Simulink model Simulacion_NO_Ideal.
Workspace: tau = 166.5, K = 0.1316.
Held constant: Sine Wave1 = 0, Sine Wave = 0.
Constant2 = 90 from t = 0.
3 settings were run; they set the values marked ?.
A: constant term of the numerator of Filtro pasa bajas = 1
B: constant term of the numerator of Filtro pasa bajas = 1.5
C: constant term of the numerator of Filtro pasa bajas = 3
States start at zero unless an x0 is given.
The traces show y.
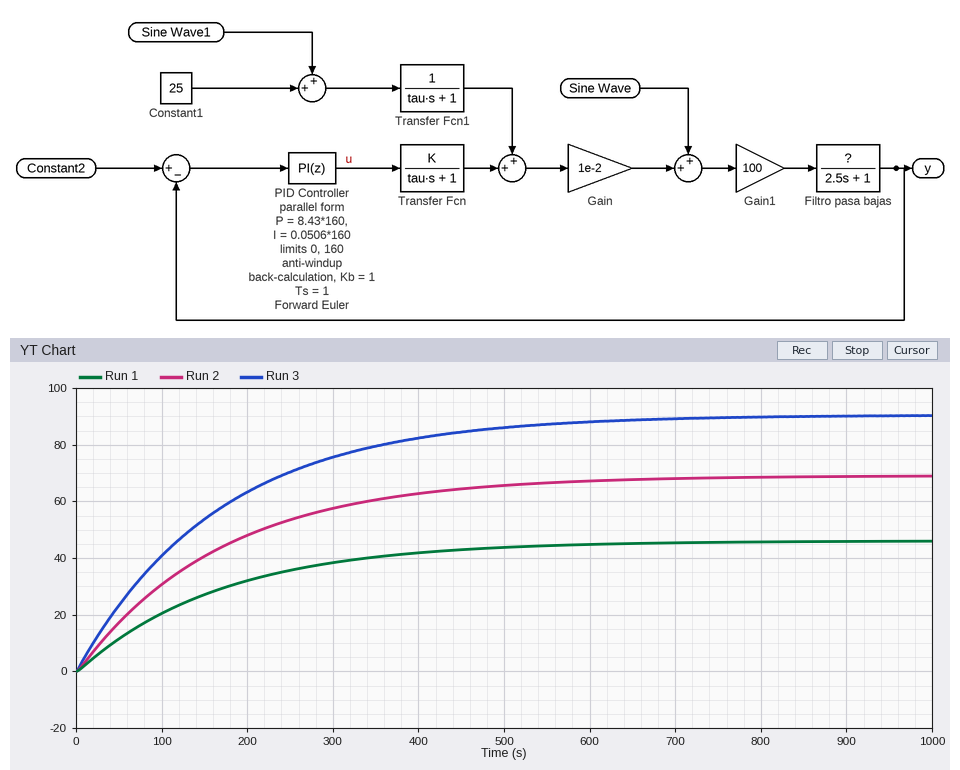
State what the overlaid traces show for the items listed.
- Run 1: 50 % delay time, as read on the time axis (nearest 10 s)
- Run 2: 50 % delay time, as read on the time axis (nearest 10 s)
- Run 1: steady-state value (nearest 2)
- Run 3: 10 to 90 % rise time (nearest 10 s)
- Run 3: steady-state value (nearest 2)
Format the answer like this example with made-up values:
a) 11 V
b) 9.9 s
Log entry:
a) 120 s
b) 120 s
c) 46
d) 360 s
e) 90
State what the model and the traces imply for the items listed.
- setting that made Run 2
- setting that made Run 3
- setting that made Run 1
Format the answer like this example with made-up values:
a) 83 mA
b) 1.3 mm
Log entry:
a) B
b) C
c) A
